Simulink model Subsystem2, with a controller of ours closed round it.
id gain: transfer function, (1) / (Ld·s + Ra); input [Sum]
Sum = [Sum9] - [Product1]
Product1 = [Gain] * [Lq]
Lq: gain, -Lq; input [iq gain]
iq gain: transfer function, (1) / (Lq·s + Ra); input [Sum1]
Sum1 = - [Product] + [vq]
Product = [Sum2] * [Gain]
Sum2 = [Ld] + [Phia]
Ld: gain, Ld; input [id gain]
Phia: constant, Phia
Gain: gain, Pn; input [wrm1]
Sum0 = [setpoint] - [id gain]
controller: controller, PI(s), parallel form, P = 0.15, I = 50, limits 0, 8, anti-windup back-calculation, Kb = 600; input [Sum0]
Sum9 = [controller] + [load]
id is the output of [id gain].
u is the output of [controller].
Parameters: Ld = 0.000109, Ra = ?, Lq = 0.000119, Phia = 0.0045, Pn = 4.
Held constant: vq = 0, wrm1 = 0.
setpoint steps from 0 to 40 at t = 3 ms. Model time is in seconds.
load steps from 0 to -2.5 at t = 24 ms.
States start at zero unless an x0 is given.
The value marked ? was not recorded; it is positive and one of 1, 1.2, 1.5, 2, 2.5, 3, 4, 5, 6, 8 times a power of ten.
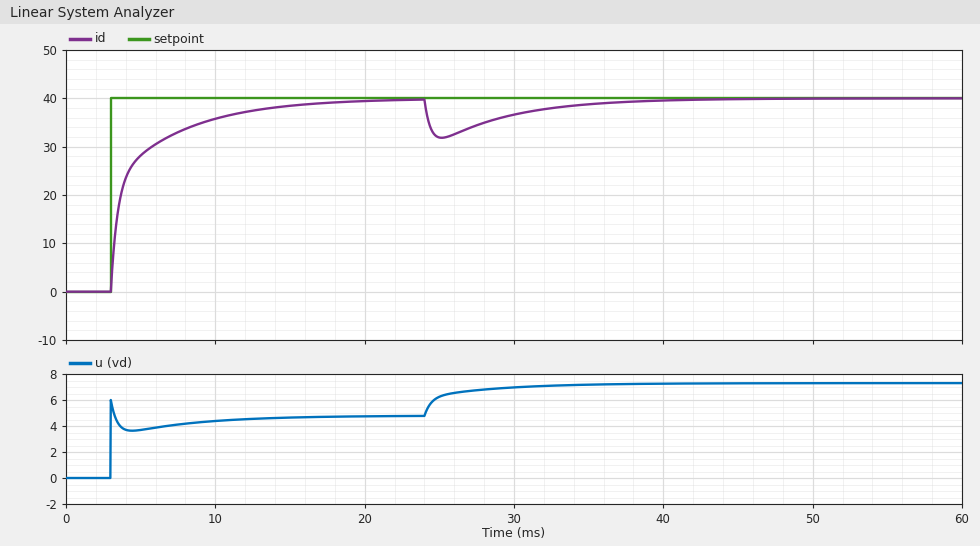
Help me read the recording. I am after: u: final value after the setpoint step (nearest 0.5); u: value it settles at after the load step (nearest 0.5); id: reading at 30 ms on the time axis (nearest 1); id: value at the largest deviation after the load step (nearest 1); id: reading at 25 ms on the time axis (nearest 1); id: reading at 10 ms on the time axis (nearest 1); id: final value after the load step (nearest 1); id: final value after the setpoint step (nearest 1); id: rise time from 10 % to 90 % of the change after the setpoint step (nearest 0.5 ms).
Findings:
5.0
7.5
37
32
32
36
40
40
7.0 ms
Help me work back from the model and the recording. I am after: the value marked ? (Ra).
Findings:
0.12
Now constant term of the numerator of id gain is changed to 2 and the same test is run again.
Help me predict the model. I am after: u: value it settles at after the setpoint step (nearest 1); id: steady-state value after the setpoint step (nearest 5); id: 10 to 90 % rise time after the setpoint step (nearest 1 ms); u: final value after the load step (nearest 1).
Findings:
2
40
4 ms
5
